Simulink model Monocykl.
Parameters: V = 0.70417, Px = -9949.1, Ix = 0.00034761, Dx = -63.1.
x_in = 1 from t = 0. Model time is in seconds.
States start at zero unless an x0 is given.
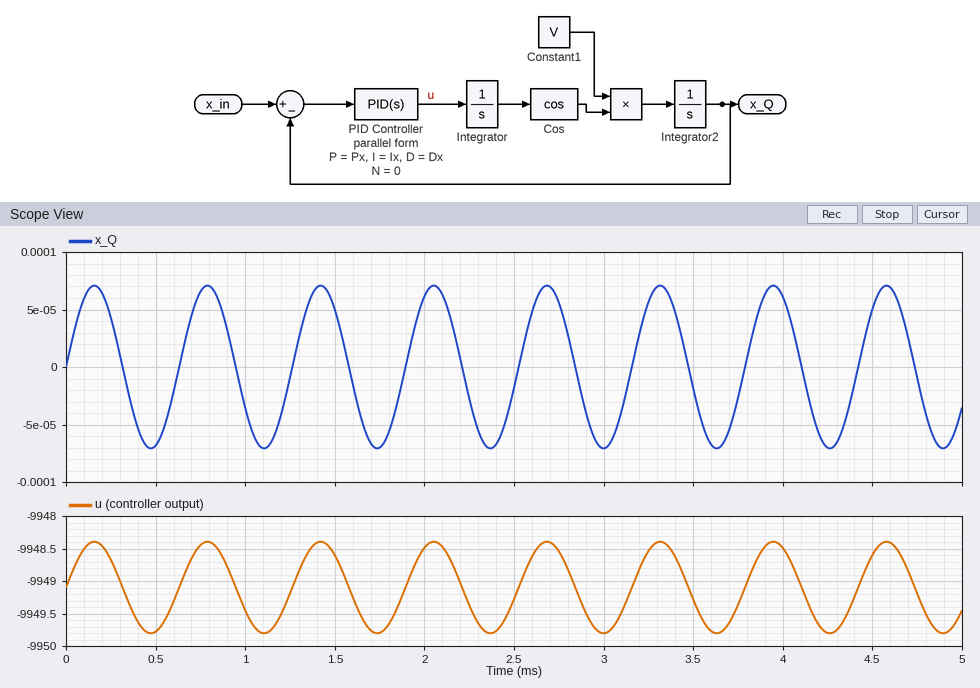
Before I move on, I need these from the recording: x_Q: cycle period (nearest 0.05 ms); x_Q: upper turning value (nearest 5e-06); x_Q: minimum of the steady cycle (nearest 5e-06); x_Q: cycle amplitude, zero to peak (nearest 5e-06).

0.65 ms
0.000070
-0.000070
0.000070
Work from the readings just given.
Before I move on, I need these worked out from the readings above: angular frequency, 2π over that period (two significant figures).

9.7 rad/ms
